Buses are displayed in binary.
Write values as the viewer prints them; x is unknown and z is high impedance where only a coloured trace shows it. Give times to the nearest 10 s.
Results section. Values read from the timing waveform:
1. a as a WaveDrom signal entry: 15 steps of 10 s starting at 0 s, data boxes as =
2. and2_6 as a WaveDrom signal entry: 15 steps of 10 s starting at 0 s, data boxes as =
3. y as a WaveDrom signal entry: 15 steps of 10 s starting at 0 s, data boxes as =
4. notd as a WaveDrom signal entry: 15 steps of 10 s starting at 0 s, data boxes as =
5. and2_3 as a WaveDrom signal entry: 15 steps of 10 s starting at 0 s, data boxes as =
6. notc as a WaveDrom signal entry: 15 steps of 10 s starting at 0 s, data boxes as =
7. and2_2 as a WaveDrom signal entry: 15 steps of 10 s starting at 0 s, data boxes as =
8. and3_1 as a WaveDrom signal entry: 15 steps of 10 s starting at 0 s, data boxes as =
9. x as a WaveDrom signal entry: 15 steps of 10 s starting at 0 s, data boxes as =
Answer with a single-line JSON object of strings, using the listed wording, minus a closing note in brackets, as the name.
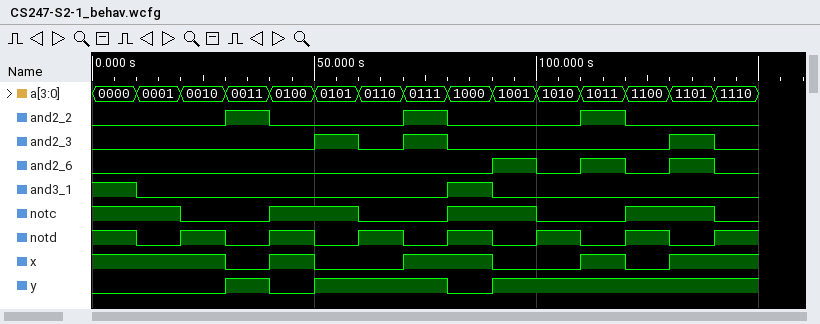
{"a as a WaveDrom signal entry: 15 steps of 10 s starting at 0 s, data boxes as =": "{name: 'a', wave: '===============', data: '0000 0001 0010 0011 0100 0101 0110 0111 1000 1001 1010 1011 1100 1101 1110'}", "and2_6 as a WaveDrom signal entry: 15 steps of 10 s starting at 0 s, data boxes as =": "{name: 'and2_6', wave: '0........101010'}", "y as a WaveDrom signal entry: 15 steps of 10 s starting at 0 s, data boxes as =": "{name: 'y', wave: '0..101..01.....'}", "notd as a WaveDrom signal entry: 15 steps of 10 s starting at 0 s, data boxes as =": "{name: 'notd', wave: '101010101010101'}", "and2_3 as a WaveDrom signal entry: 15 steps of 10 s starting at 0 s, data boxes as =": "{name: 'and2_3', wave: '0....1010....10'}", "notc as a WaveDrom signal entry: 15 steps of 10 s starting at 0 s, data boxes as =": "{name: 'notc', wave: '1.0.1.0.1.0.1.0'}", "and2_2 as a WaveDrom signal entry: 15 steps of 10 s starting at 0 s, data boxes as =": "{name: 'and2_2', wave: '0..10..10..10..'}", "and3_1 as a WaveDrom signal entry: 15 steps of 10 s starting at 0 s, data boxes as =": "{name: 'and3_1', wave: '10......10.....'}", "x as a WaveDrom signal entry: 15 steps of 10 s starting at 0 s, data boxes as =": "{name: 'x', wave: '1..010.1.0.101.'}"}
